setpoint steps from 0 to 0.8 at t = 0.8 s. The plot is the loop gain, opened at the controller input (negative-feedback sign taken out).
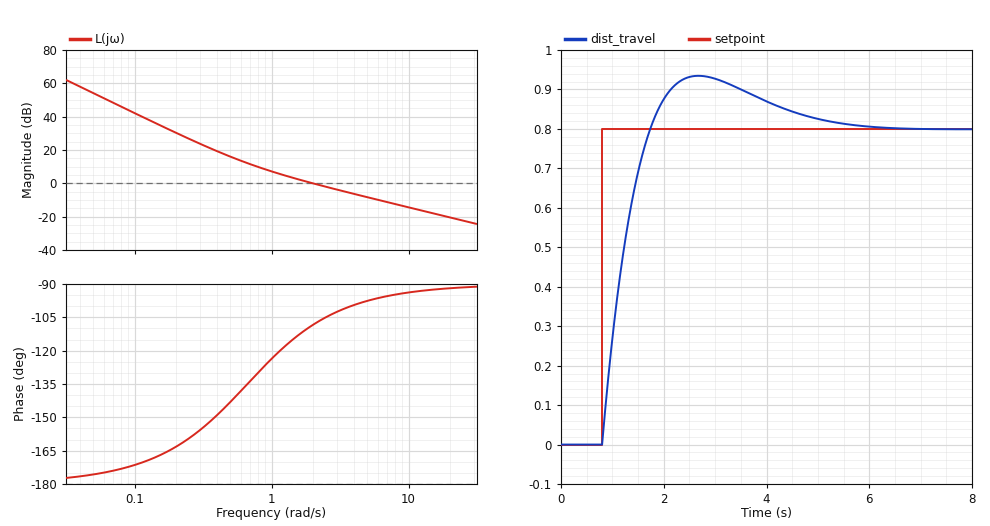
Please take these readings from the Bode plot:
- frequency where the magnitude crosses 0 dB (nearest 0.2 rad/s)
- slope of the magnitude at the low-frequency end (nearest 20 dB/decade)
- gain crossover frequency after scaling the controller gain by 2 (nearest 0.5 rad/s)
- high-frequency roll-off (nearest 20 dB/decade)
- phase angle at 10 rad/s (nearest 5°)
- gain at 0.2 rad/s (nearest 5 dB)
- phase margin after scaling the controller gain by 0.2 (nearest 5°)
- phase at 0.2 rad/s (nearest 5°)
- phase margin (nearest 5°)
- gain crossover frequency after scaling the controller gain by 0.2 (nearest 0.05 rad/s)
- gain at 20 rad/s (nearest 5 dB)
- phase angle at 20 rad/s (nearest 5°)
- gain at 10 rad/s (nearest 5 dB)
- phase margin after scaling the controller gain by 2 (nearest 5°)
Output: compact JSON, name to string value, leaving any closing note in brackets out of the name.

{"frequency where the magnitude crosses 0 dB": "2.0 rad/s", "slope of the magnitude at the low-frequency end": "-40 dB/decade", "gain crossover frequency after scaling the controller gain by 2": "4.0 rad/s", "high-frequency roll-off": "-20 dB/decade", "phase angle at 10 rad/s": "-95°", "gain at 0.2 rad/s": "30 dB", "phase margin after scaling the controller gain by 0.2": "40°", "phase at 0.2 rad/s": "-165°", "phase margin": "70°", "gain crossover frequency after scaling the controller gain by 0.2": "0.60 rad/s", "gain at 20 rad/s": "-20 dB", "phase angle at 20 rad/s": "-90°", "gain at 10 rad/s": "-15 dB", "phase margin after scaling the controller gain by 2": "80°"}
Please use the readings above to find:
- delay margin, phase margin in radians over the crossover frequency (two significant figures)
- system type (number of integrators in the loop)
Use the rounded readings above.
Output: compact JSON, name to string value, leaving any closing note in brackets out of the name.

{"delay margin, phase margin in radians over the crossover frequency": "0.61 s", "system type": "2"}
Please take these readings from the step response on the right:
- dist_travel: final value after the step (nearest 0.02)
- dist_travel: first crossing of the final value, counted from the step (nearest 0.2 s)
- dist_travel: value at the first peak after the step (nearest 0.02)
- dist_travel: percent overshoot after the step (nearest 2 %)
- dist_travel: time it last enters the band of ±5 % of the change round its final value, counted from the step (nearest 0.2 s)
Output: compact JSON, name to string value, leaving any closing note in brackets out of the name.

{"dist_travel: final value after the step": "0.80", "dist_travel: first crossing of the final value, counted from the step": "1.0 s", "dist_travel: value at the first peak after the step": "0.94", "dist_travel: percent overshoot after the step": "16 %", "dist_travel: time it last enters the band of ±5 % of the change round its final value, counted from the step": "3.8 s"}
